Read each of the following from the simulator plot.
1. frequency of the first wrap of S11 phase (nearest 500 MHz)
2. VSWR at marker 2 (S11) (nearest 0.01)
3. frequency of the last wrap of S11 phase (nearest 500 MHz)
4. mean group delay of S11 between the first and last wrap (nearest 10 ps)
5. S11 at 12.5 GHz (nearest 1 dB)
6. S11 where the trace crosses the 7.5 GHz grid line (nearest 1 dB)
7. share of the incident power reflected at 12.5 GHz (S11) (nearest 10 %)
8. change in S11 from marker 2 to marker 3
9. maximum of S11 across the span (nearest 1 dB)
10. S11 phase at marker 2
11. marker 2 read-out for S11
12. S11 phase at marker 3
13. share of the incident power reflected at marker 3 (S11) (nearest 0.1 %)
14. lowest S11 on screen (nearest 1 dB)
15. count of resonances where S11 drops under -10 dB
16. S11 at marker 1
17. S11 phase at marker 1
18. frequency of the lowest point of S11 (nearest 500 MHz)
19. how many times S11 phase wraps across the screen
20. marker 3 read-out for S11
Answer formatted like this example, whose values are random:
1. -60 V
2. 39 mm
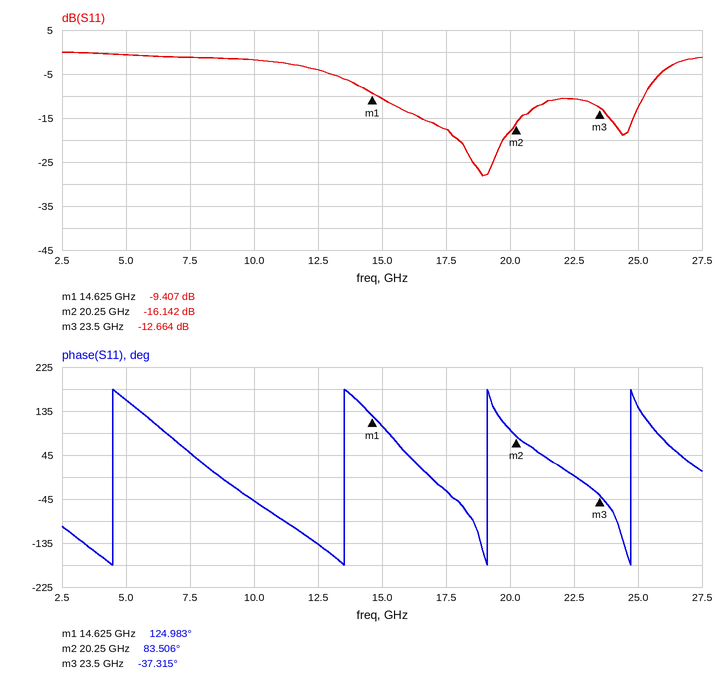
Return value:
1. 4.5 GHz
2. 1.37
3. 24.5 GHz
4. 150 ps
5. -4 dB
6. -1 dB
7. 40 %
8. 3.478 dB
9. 0 dB
10. 83.506°
11. -16.142 dB
12. -37.315°
13. 5.4 %
14. -28 dB
15. 2
16. -9.407 dB
17. 124.983°
18. 19.0 GHz
19. 4
20. -12.664 dB
